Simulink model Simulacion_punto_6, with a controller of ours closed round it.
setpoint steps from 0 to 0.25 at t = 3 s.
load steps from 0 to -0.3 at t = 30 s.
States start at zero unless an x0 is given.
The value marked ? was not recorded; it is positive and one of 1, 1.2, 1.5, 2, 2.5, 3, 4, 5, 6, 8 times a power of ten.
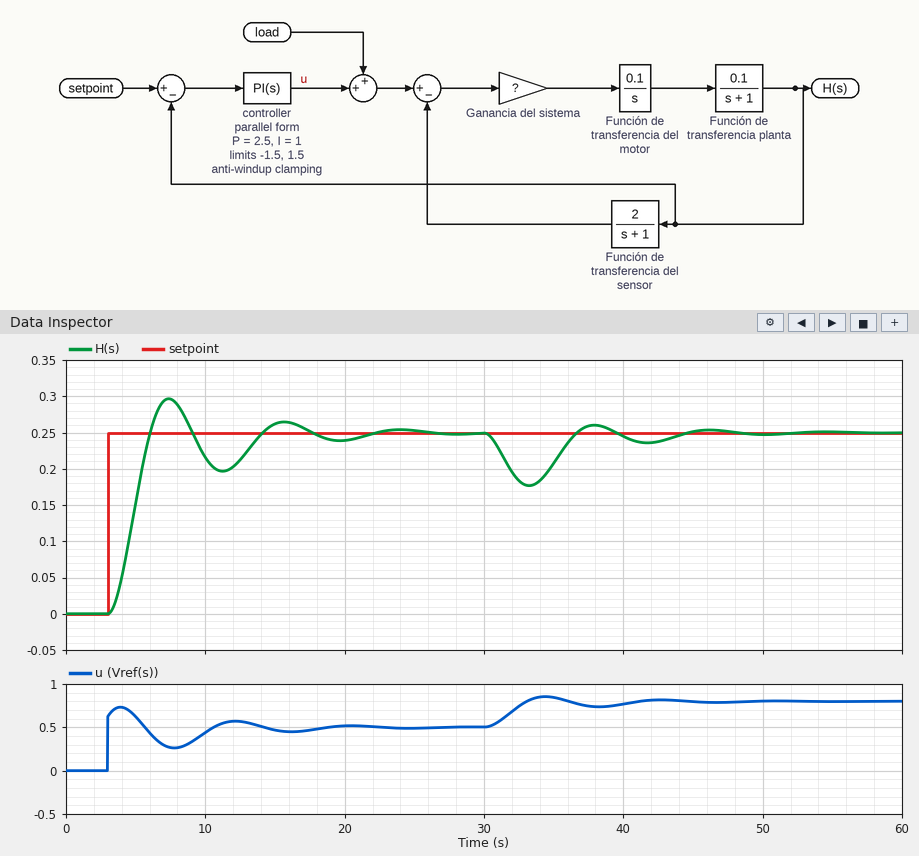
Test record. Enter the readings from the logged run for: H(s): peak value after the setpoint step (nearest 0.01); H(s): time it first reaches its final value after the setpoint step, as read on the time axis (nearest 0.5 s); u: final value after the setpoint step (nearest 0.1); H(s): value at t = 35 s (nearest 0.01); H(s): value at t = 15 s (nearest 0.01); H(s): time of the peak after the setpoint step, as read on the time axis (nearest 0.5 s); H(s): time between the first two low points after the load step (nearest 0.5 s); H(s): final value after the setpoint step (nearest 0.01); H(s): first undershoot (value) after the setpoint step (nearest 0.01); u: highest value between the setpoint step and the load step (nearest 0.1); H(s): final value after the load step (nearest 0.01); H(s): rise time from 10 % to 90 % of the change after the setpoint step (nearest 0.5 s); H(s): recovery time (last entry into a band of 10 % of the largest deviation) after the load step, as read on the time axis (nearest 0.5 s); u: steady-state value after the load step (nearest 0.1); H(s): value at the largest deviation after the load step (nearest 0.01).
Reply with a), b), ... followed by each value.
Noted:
a) 0.30
b) 6.0 s
c) 0.5
d) 0.21
e) 0.26
f) 7.5 s
g) 8.5 s
h) 0.25
i) 0.20
j) 0.7
k) 0.25
l) 2.0 s
m) 43.5 s
n) 0.8
o) 0.18
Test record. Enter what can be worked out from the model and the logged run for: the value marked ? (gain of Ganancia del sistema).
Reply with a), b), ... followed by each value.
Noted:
a) 20
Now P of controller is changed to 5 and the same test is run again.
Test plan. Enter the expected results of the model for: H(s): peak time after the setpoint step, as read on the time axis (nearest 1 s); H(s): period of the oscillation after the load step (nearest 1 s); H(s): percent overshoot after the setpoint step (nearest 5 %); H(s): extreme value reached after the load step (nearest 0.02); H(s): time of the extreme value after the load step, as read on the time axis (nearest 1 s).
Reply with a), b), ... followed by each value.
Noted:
a) 6 s
b) 6 s
c) 20 %
d) 0.20
e) 33 s
